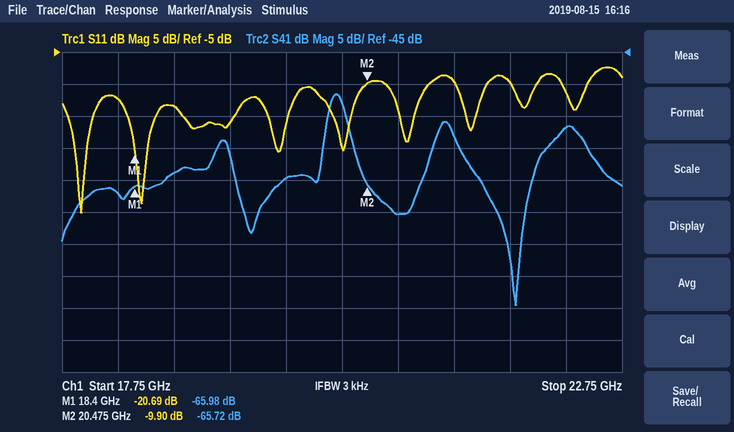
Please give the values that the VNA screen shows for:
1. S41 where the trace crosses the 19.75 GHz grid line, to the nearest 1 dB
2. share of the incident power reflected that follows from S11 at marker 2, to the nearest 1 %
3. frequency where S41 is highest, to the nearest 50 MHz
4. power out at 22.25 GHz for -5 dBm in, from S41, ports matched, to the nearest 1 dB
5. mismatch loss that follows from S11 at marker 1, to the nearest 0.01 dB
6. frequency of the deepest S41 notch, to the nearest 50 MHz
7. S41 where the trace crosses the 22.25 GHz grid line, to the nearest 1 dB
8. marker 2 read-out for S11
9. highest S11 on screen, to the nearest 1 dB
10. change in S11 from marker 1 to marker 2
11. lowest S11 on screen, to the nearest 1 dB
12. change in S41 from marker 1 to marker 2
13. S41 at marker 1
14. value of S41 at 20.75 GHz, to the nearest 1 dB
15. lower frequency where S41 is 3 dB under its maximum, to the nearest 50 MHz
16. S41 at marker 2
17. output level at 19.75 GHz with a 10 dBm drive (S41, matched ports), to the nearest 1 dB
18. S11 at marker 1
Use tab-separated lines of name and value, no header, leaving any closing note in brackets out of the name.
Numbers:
S41 where the trace crosses the 19.75 GHz grid line, to the nearest 1 dB	-65 dB
share of the incident power reflected that follows from S11 at marker 2, to the nearest 1 %	10 %
frequency where S41 is highest, to the nearest 50 MHz	20.20 GHz
power out at 22.25 GHz for -5 dBm in, from S41, ports matched, to the nearest 1 dB	-62 dBm
mismatch loss that follows from S11 at marker 1, to the nearest 0.01 dB	0.04 dB
frequency of the deepest S41 notch, to the nearest 50 MHz	21.80 GHz
S41 where the trace crosses the 22.25 GHz grid line, to the nearest 1 dB	-57 dB
marker 2 read-out for S11	-9.90 dB
highest S11 on screen, to the nearest 1 dB	-7 dB
change in S11 from marker 1 to marker 2	10.79 dB
lowest S11 on screen, to the nearest 1 dB	-30 dB
change in S41 from marker 1 to marker 2	0.26 dB
S41 at marker 1	-65.98 dB
value of S41 at 20.75 GHz, to the nearest 1 dB	-70 dB
lower frequency where S41 is 3 dB under its maximum, to the nearest 50 MHz	20.15 GHz
S41 at marker 2	-65.72 dB
output level at 19.75 GHz with a 10 dBm drive (S41, matched ports), to the nearest 1 dB	-55 dBm
S11 at marker 1	-20.69 dB
